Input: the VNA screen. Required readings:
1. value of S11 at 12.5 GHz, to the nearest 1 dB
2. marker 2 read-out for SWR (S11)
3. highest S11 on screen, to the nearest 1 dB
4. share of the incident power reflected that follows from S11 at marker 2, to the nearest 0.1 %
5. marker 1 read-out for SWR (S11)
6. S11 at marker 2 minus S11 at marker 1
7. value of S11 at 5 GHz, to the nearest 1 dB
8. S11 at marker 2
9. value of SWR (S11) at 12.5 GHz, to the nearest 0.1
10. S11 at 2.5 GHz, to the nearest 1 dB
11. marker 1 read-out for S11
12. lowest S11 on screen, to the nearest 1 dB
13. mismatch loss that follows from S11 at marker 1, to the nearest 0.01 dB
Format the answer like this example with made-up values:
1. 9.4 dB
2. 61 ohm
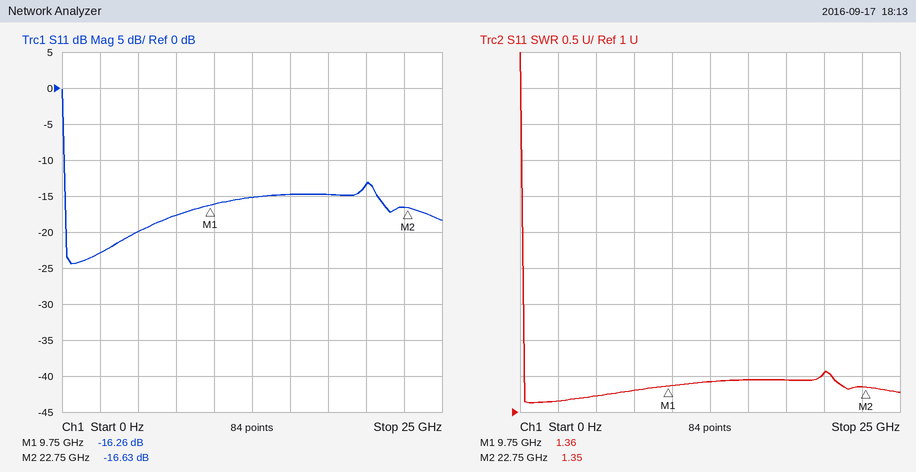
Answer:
1. -15 dB
2. 1.35
3. 0 dB
4. 2.2 %
5. 1.36
6. -0.37 dB
7. -20 dB
8. -16.63 dB
9. 1.4
10. -23 dB
11. -16.26 dB
12. -24 dB
13. 0.10 dB
